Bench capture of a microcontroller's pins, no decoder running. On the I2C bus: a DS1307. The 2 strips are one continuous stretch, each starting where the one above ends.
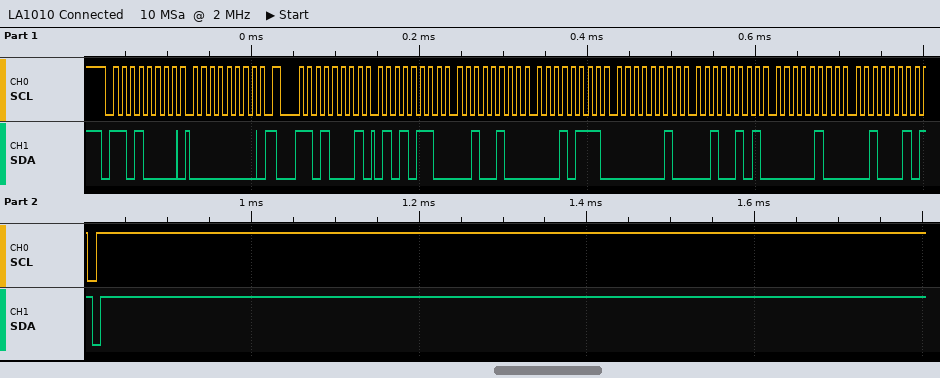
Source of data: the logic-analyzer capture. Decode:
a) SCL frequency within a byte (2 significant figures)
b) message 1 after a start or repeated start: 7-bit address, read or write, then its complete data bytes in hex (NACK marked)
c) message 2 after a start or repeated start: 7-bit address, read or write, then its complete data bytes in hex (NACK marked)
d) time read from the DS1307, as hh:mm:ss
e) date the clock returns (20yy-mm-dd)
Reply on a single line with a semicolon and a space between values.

100 kHz; 0x68 write: 00; 0x68 read: 56 24 17 02 25 04 22 NACK; 17:24:56; 2022-04-25
